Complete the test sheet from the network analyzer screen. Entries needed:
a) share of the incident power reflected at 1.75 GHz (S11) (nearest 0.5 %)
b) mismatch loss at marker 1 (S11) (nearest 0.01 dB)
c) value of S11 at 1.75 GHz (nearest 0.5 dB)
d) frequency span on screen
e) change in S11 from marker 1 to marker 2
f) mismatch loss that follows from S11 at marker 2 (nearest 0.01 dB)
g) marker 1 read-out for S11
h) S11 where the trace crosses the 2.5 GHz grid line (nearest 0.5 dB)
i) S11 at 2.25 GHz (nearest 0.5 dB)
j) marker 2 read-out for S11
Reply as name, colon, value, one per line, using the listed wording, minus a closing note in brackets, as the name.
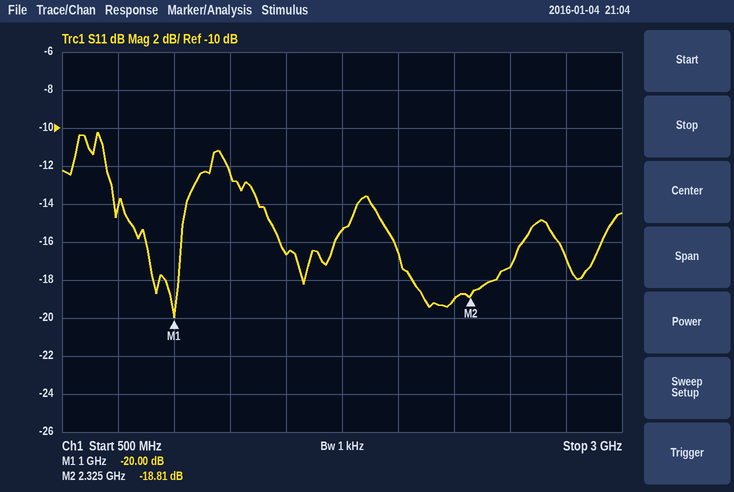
share of the incident power reflected at 1.75 GHz (S11): 3.0 %
mismatch loss at marker 1 (S11): 0.04 dB
value of S11 at 1.75 GHz: -15.5 dB
frequency span on screen: 2.5 GHz
change in S11 from marker 1 to marker 2: 1.19 dB
mismatch loss that follows from S11 at marker 2: 0.06 dB
marker 1 read-out for S11: -20.00 dB
S11 where the trace crosses the 2.5 GHz grid line: -17.5 dB
S11 at 2.25 GHz: -19.0 dB
marker 2 read-out for S11: -18.81 dB
